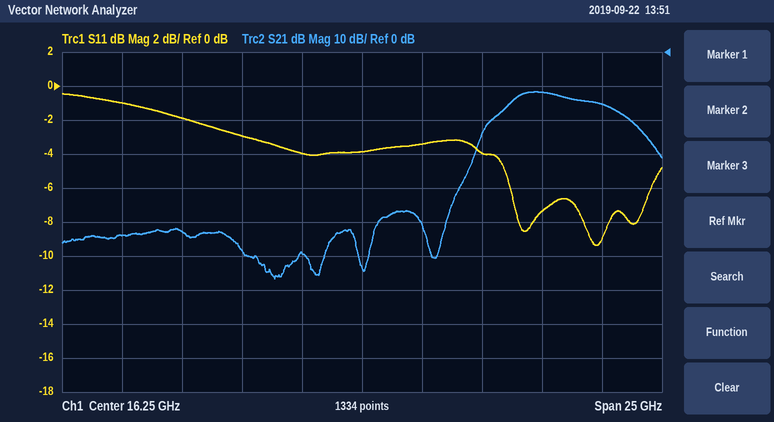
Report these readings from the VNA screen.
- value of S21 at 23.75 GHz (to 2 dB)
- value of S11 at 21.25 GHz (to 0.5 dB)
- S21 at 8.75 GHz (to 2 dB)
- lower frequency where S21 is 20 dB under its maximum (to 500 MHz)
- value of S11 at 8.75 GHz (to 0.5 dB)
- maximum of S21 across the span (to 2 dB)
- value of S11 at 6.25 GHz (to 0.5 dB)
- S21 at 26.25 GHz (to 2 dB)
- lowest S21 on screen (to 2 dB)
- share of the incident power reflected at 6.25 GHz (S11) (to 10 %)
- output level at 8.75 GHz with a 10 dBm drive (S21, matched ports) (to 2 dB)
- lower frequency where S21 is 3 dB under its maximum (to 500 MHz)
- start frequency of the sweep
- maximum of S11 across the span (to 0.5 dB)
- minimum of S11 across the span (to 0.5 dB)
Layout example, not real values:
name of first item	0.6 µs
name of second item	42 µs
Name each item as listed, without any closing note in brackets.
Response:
value of S21 at 23.75 GHz	-12 dB
value of S11 at 21.25 GHz	-4.0 dB
S21 at 8.75 GHz	-52 dB
lower frequency where S21 is 20 dB under its maximum	21.0 GHz
value of S11 at 8.75 GHz	-2.0 dB
maximum of S21 across the span	-12 dB
value of S11 at 6.25 GHz	-1.0 dB
S21 at 26.25 GHz	-16 dB
lowest S21 on screen	-66 dB
share of the incident power reflected at 6.25 GHz (S11)	80 %
output level at 8.75 GHz with a 10 dBm drive (S21, matched ports)	-42 dBm
lower frequency where S21 is 3 dB under its maximum	22.5 GHz
start frequency of the sweep	3.75 GHz
maximum of S11 across the span	-0.5 dB
minimum of S11 across the span	-9.5 dB
